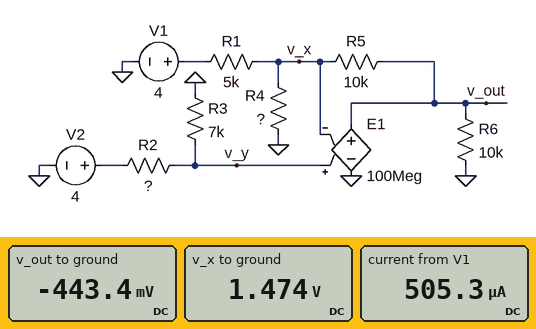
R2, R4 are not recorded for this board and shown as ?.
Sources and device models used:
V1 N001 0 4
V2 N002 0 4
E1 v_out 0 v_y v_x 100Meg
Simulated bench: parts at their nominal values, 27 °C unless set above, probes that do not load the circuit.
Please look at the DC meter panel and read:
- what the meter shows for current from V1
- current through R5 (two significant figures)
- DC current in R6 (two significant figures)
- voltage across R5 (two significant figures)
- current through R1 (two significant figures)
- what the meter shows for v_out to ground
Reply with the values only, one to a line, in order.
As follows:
505.3 µA
190 µA
44 µA
1.9 V
510 µA
-443.4 mV
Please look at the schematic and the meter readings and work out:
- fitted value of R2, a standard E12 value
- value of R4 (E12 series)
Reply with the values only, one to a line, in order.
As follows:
12 kΩ
4.7 kΩ
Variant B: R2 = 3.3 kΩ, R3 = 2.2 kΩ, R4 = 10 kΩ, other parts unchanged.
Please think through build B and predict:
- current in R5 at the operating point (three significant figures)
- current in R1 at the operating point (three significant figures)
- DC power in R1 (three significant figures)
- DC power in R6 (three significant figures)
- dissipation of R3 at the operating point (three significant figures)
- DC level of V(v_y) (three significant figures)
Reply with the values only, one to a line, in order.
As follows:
320 µA
480 µA
1.15 mW
256 µW
1.16 mW
1.60 V
